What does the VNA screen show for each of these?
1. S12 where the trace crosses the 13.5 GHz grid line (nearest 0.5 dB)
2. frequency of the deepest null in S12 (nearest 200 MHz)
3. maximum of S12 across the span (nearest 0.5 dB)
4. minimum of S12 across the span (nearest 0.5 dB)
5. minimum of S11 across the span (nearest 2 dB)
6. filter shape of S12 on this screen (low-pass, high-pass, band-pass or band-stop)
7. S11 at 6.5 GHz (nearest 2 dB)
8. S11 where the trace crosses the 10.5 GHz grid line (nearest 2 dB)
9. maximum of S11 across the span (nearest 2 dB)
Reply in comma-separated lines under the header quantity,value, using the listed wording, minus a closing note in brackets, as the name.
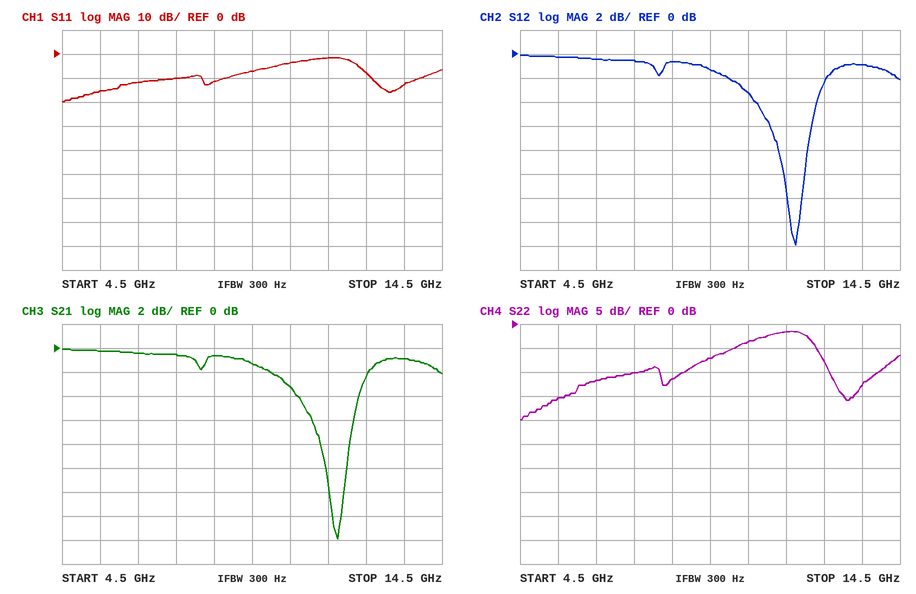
quantity,value
S12 where the trace crosses the 13.5 GHz grid line,-1.0 dB
frequency of the deepest null in S12,11.8 GHz
maximum of S12 across the span,0.0 dB
minimum of S12 across the span,-16.0 dB
minimum of S11 across the span,-20 dB
filter shape of S12 on this screen,band-stop
S11 at 6.5 GHz,-12 dB
S11 where the trace crosses the 10.5 GHz grid line,-4 dB
maximum of S11 across the span,-2 dB
